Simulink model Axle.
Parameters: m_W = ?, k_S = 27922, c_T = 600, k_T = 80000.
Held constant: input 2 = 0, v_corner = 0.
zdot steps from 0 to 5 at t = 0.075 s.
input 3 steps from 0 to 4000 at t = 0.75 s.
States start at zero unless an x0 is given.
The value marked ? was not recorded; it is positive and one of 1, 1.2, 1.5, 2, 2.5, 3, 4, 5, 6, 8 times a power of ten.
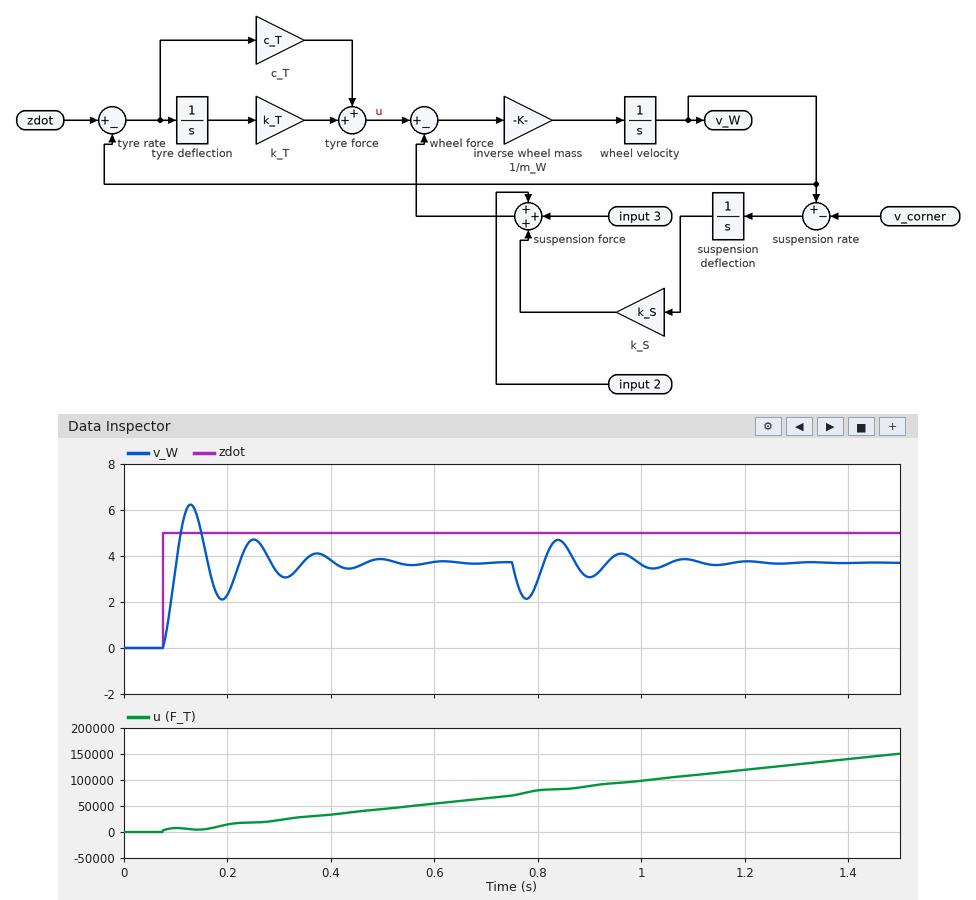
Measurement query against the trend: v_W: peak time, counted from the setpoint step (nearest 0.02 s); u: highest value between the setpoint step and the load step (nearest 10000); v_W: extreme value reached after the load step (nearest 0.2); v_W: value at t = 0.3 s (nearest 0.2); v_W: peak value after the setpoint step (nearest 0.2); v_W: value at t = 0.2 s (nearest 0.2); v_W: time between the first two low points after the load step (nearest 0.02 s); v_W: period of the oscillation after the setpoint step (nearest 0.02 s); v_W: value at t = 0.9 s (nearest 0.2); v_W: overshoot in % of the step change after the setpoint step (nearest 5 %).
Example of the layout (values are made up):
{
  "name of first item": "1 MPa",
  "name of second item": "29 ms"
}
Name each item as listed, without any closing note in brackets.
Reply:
{
  "v_W: peak time, counted from the setpoint step": "0.06 s",
  "u: highest value between the setpoint step and the load step": "70000",
  "v_W: extreme value reached after the load step": "2.2",
  "v_W: value at t = 0.3 s": "3.2",
  "v_W: peak value after the setpoint step": "6.2",
  "v_W: value at t = 0.2 s": "2.4",
  "v_W: time between the first two low points after the load step": "0.12 s",
  "v_W: period of the oscillation after the setpoint step": "0.12 s",
  "v_W: value at t = 0.9 s": "3.0",
  "v_W: overshoot in % of the step change after the setpoint step": "70 %"
}
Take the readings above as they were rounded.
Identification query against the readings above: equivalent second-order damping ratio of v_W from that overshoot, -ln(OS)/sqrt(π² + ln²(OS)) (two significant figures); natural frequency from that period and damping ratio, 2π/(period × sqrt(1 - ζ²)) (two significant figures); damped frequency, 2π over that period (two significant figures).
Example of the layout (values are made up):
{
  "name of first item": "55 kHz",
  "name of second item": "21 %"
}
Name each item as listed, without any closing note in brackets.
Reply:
{
  "equivalent second-order damping ratio of v_W from that overshoot, -ln(OS)/sqrt(π² + ln²(OS))": "0.11",
  "natural frequency from that period and damping ratio, 2π/(period × sqrt(1 - ζ²))": "53 rad/s",
  "damped frequency, 2π over that period": "52 rad/s"
}
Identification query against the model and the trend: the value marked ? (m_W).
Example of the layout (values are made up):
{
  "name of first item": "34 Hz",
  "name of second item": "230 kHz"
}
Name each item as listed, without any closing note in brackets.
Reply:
{
  "the value marked ?": "40"
}
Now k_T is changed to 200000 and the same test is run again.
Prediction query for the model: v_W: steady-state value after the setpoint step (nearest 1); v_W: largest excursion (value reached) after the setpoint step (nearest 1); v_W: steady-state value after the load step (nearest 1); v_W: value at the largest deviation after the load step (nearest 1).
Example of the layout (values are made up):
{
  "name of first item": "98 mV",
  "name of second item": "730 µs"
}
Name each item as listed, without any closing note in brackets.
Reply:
{
  "v_W: steady-state value after the setpoint step": "4",
  "v_W: largest excursion (value reached) after the setpoint step": "8",
  "v_W: steady-state value after the load step": "4",
  "v_W: value at the largest deviation after the load step": "3"
}
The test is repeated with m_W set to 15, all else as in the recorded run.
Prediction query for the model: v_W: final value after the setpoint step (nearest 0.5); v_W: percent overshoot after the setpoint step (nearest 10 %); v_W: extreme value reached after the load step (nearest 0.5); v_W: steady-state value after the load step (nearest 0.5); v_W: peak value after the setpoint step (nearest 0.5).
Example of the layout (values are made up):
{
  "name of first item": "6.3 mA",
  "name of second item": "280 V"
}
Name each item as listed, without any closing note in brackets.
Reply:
{
  "v_W: final value after the setpoint step": "3.5",
  "v_W: percent overshoot after the setpoint step": "60 %",
  "v_W: extreme value reached after the load step": "1.5",
  "v_W: steady-state value after the load step": "3.5",
  "v_W: peak value after the setpoint step": "6.0"
}
